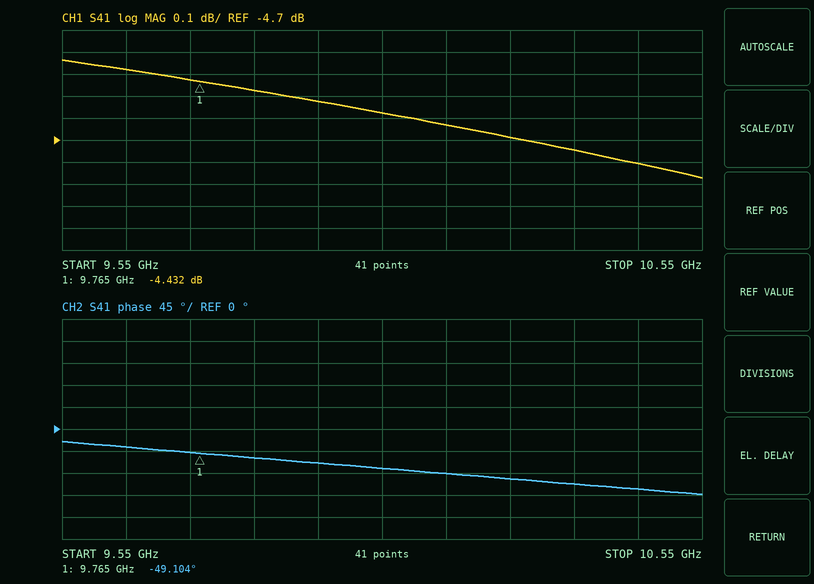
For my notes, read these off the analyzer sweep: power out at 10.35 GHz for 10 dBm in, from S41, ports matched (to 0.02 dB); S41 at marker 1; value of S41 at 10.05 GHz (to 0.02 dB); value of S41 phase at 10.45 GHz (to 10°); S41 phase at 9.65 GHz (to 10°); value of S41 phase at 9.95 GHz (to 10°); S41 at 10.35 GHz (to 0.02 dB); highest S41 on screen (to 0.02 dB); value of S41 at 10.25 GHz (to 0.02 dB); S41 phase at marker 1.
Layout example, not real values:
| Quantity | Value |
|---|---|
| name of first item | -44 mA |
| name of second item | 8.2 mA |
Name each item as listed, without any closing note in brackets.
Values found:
| Quantity | Value |
|---|---|
| power out at 10.35 GHz for 10 dBm in, from S41, ports matched | 5.26 dBm |
| S41 at marker 1 | -4.432 dB |
| value of S41 at 10.05 GHz | -4.58 dB |
| value of S41 phase at 10.45 GHz | -120° |
| S41 phase at 9.65 GHz | -40° |
| value of S41 phase at 9.95 GHz | -70° |
| S41 at 10.35 GHz | -4.74 dB |
| highest S41 on screen | -4.34 dB |
| value of S41 at 10.25 GHz | -4.68 dB |
| S41 phase at marker 1 | -49.104° |
